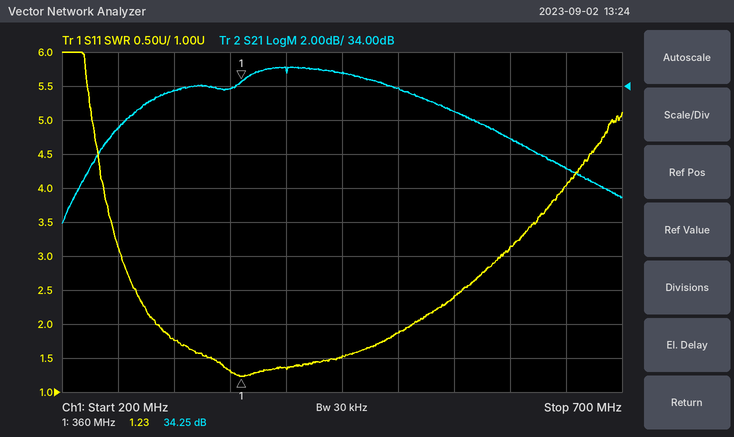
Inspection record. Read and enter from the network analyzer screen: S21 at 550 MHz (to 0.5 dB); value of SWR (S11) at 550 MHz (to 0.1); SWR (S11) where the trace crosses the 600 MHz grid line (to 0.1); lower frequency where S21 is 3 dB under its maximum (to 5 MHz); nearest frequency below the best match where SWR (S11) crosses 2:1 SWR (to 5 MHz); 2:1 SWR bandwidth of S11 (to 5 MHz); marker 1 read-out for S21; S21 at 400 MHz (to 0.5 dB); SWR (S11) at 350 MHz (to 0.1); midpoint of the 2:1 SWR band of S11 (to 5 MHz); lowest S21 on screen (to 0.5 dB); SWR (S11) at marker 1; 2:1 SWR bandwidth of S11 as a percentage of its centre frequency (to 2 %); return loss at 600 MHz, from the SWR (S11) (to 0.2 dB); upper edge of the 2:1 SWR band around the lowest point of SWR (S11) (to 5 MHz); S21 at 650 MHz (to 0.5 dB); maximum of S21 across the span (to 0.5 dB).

32.5 dB
2.4
3.1
260 MHz
285 MHz
230 MHz
34.25 dB
35.0 dB
1.3
400 MHz
26.0 dB
1.23
58 %
5.8 dB
515 MHz
29.0 dB
35.0 dB
